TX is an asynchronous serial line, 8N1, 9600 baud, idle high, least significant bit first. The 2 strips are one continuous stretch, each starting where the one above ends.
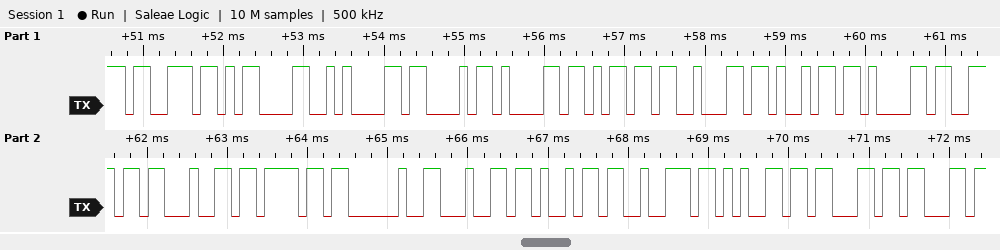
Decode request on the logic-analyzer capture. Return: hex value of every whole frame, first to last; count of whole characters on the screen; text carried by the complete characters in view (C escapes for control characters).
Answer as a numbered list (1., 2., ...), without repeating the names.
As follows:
1. 73 0D 0A 43 61 6D 62 69 61 6E 64 6F 20 64 69 72 65 63 63
2. 19
3. "s\r\nCambiando direcc"
